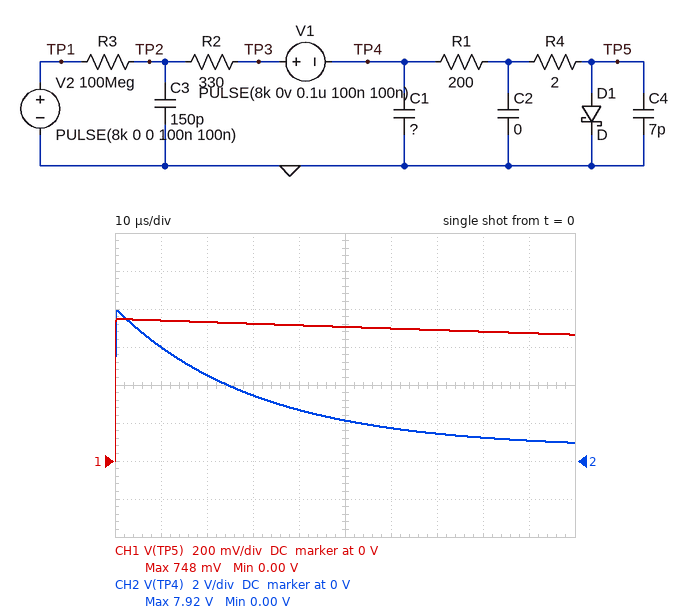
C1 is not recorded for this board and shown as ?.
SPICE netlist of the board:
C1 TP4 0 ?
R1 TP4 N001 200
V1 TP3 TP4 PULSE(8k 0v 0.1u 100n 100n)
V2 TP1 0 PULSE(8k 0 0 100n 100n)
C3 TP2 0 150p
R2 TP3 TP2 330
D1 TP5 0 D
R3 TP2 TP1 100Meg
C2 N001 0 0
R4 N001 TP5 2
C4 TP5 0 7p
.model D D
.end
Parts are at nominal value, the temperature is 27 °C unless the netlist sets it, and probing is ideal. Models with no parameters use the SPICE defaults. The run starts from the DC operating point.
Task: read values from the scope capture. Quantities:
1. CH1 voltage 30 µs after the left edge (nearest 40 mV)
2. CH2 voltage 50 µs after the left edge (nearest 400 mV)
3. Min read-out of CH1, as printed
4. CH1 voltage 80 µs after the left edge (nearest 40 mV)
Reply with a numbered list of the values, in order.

1. 720 mV
2. 2.0 V
3. 0.00 V
4. 680 mV
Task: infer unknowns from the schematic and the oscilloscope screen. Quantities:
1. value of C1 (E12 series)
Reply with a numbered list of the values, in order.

1. 150 nF
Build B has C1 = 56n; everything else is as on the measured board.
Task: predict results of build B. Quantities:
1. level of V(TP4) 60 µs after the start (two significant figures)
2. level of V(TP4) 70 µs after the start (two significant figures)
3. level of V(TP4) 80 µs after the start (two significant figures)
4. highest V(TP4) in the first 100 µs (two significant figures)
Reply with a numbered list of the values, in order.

1. 770 mV
2. 690 mV
3. 650 mV
4. 21 V
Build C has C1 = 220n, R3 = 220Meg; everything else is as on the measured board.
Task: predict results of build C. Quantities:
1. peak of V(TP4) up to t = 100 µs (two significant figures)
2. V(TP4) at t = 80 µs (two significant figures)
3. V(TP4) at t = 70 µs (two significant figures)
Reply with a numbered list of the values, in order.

1. 5.4 V
2. 1.5 V
3. 1.7 V
